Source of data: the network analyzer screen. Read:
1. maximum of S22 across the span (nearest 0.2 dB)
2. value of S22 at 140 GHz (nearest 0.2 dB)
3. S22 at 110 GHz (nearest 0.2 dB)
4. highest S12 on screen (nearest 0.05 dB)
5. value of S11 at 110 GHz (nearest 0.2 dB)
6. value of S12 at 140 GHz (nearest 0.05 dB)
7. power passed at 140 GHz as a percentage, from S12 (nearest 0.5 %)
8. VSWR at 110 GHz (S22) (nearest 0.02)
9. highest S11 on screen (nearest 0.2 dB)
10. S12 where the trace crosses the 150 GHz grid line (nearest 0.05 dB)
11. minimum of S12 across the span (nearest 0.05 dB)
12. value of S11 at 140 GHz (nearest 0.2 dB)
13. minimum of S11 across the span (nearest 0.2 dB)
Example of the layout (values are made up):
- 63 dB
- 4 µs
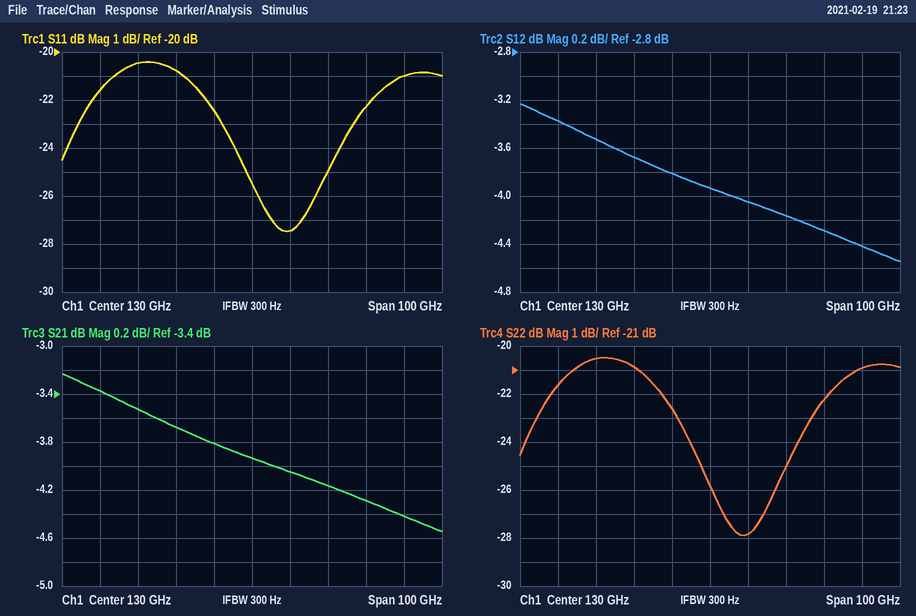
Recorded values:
- -20.4 dB
- -27.8 dB
- -20.8 dB
- -3.25 dB
- -20.8 dB
- -4.05 dB
- 39.5 %
- 1.20
- -20.4 dB
- -4.15 dB
- -4.55 dB
- -27.4 dB
- -27.4 dB
